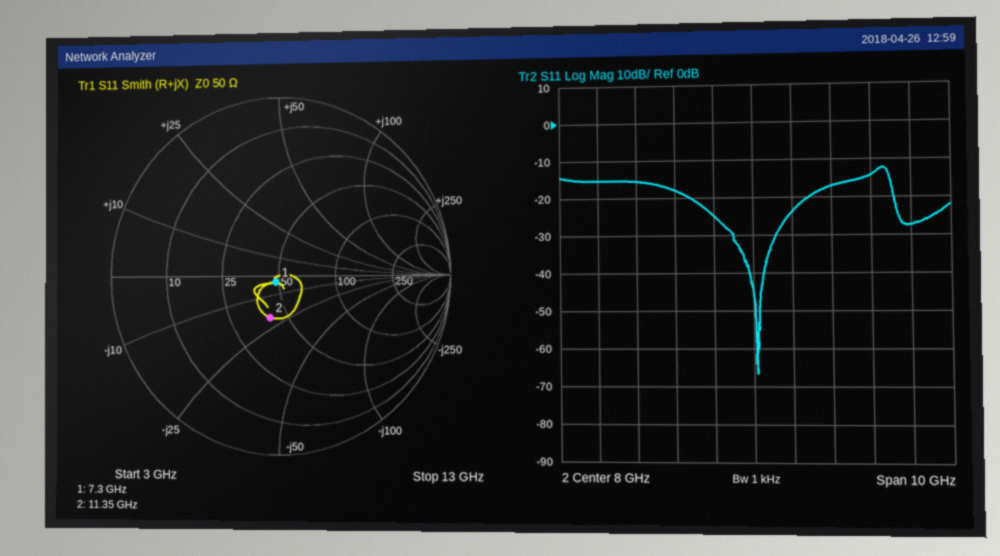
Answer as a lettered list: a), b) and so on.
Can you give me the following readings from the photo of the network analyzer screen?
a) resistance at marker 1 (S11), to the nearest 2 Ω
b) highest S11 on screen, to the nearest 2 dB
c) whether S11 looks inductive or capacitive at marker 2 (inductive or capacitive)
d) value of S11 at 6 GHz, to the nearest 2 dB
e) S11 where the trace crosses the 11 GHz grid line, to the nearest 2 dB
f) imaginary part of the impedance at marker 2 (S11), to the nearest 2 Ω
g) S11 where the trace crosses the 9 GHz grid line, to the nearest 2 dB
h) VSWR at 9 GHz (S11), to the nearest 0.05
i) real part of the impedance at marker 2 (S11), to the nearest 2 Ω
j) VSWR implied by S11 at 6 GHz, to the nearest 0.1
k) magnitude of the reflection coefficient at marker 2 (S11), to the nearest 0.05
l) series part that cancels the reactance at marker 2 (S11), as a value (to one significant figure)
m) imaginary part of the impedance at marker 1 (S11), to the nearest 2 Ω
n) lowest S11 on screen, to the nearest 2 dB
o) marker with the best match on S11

a) 48 Ω
b) -12 dB
c) capacitive
d) -18 dB
e) -14 dB
f) -20 Ω
g) -24 dB
h) 1.15
i) 40 Ω
j) 1.3
k) 0.25
l) 300 pH
m) -4 Ω
n) -66 dB
o) marker 1
